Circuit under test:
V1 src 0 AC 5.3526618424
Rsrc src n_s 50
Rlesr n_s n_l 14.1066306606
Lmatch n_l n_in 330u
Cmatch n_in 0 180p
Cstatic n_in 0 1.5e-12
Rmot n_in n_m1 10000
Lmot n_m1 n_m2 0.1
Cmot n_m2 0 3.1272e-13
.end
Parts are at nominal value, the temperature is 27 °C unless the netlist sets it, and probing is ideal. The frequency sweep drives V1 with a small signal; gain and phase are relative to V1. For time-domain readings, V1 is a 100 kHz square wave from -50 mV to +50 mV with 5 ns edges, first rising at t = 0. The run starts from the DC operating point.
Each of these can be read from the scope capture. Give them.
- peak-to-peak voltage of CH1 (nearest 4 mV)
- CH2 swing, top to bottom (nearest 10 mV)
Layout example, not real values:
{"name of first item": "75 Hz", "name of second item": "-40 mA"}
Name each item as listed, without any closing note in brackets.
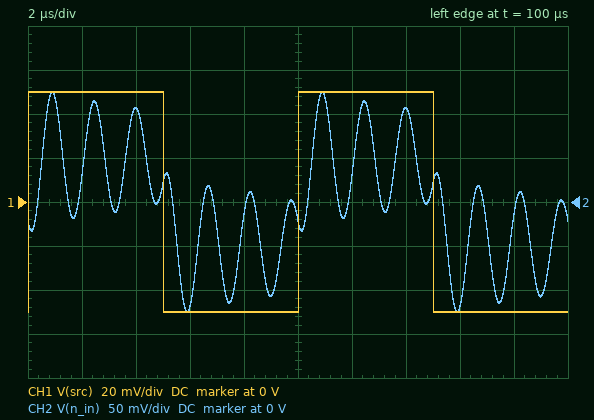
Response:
{"peak-to-peak voltage of CH1": "100 mV", "CH2 swing, top to bottom": "250 mV"}
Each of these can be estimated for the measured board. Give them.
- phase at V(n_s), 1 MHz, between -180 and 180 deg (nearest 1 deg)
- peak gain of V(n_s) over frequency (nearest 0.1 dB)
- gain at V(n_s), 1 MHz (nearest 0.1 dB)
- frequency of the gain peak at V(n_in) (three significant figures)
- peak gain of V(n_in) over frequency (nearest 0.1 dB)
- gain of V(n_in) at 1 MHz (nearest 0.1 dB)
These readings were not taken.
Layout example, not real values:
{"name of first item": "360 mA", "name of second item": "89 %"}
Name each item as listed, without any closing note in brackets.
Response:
{"phase at V(n_s), 1 MHz, between -180 and 180 deg": "2 deg", "peak gain of V(n_s) over frequency": "0 dB", "gain at V(n_s), 1 MHz": "0 dB", "frequency of the gain peak at V(n_in)": "649 kHz", "peak gain of V(n_in) over frequency": "26.4 dB", "gain of V(n_in) at 1 MHz": "-2.6 dB"}
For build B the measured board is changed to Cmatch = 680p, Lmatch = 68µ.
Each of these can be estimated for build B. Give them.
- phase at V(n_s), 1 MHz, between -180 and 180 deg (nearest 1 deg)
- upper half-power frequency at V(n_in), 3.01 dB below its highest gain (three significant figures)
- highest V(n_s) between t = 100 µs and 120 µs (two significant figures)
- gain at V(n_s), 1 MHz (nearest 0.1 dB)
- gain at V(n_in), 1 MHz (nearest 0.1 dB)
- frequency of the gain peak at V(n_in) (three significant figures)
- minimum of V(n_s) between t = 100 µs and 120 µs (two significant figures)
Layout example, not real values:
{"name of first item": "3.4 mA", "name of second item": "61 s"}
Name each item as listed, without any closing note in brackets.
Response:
{"phase at V(n_s), 1 MHz, between -180 and 180 deg": "14 deg", "upper half-power frequency at V(n_in), 3.01 dB below its highest gain": "803 kHz", "highest V(n_s) between t = 100 µs and 120 µs": "60 mV", "gain at V(n_s), 1 MHz": "-0.4 dB", "gain at V(n_in), 1 MHz": "1.2 dB", "frequency of the gain peak at V(n_in)": "731 kHz", "minimum of V(n_s) between t = 100 µs and 120 µs": "-60 mV"}
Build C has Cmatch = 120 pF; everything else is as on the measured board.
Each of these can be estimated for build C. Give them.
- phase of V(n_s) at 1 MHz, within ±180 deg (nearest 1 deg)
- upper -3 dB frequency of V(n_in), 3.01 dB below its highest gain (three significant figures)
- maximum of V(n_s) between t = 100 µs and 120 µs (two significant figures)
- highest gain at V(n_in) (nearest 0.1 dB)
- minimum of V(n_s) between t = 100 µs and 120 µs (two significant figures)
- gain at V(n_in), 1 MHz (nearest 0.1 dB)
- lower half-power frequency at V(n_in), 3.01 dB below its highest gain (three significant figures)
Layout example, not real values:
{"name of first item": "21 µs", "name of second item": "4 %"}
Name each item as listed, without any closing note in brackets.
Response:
{"phase of V(n_s) at 1 MHz, within ±180 deg": "4 deg", "upper -3 dB frequency of V(n_in), 3.01 dB below its highest gain": "805 kHz", "maximum of V(n_s) between t = 100 µs and 120 µs": "52 mV", "highest gain at V(n_in)": "28.0 dB", "minimum of V(n_s) between t = 100 µs and 120 µs": "-52 mV", "gain at V(n_in), 1 MHz": "4.9 dB", "lower half-power frequency at V(n_in), 3.01 dB below its highest gain": "775 kHz"}
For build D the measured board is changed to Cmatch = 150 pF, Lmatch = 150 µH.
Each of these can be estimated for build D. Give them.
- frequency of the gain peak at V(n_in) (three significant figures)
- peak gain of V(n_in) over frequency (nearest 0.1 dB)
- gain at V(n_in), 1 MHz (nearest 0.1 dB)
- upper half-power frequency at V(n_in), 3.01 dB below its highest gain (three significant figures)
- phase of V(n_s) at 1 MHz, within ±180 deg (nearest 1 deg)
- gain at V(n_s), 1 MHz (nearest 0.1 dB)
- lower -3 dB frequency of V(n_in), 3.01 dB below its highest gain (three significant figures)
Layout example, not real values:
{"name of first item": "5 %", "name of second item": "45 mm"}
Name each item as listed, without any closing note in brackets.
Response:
{"frequency of the gain peak at V(n_in)": "1.06 MHz", "peak gain of V(n_in) over frequency": "23.8 dB", "gain at V(n_in), 1 MHz": "18.0 dB", "upper half-power frequency at V(n_in), 3.01 dB below its highest gain": "1.09 MHz", "phase of V(n_s) at 1 MHz, within ±180 deg": "-22 deg", "gain at V(n_s), 1 MHz": "-1.1 dB", "lower -3 dB frequency of V(n_in), 3.01 dB below its highest gain": "1.02 MHz"}
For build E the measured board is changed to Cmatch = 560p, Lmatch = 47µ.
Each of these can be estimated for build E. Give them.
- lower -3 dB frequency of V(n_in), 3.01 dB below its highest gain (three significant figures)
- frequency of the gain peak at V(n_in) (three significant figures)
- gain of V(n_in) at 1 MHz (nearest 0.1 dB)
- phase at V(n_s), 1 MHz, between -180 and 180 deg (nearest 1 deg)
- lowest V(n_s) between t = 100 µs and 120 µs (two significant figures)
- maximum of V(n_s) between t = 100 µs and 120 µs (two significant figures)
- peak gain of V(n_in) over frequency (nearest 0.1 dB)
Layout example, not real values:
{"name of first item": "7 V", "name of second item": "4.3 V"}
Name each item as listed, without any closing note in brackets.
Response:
{"lower -3 dB frequency of V(n_in), 3.01 dB below its highest gain": "850 kHz", "frequency of the gain peak at V(n_in)": "970 kHz", "gain of V(n_in) at 1 MHz": "12.8 dB", "phase at V(n_s), 1 MHz, between -180 and 180 deg": "28 deg", "lowest V(n_s) between t = 100 µs and 120 µs": "-60 mV", "maximum of V(n_s) between t = 100 µs and 120 µs": "60 mV", "peak gain of V(n_in) over frequency": "13.1 dB"}
